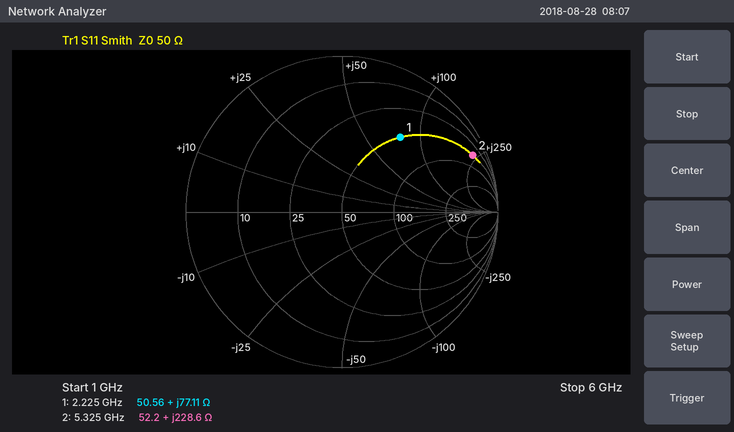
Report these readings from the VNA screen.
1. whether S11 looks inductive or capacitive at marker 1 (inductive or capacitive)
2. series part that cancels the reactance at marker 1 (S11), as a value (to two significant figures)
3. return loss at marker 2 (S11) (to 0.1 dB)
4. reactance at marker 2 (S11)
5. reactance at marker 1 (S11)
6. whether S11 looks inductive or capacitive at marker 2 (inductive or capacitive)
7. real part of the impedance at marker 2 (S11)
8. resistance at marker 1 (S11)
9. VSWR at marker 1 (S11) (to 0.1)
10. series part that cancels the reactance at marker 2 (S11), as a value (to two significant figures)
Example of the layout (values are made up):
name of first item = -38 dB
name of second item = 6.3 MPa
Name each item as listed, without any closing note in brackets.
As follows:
whether S11 looks inductive or capacitive at marker 1 = inductive
series part that cancels the reactance at marker 1 (S11), as a value = 930 fF
return loss at marker 2 (S11) = 0.8 dB
reactance at marker 2 = +228.6 Ω
reactance at marker 1 = +77.11 Ω
whether S11 looks inductive or capacitive at marker 2 = inductive
real part of the impedance at marker 2 = 52.2 Ω
resistance at marker 1 = 50.56 Ω
VSWR at marker 1 (S11) = 4.1
series part that cancels the reactance at marker 2 (S11), as a value = 130 fF
